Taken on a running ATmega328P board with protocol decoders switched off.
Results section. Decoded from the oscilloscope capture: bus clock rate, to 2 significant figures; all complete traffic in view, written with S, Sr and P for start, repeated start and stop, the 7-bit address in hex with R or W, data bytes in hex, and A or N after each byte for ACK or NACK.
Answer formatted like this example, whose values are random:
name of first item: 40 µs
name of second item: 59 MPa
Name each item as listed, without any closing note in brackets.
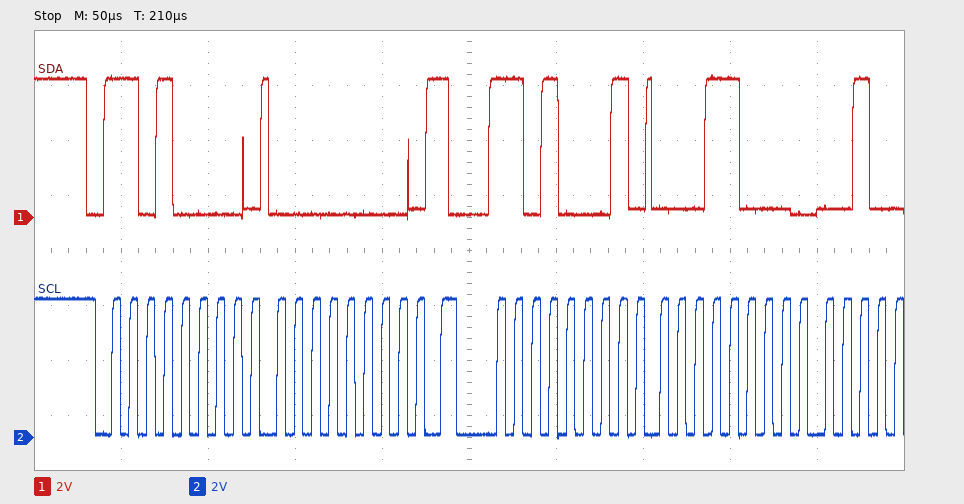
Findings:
bus clock rate, to 2 significant figures: 100 kHz
all complete traffic in view, written with S, Sr and P for start, repeated start and stop, the 7-bit address in hex with R or W, data bytes in hex, and A or N after each byte for ACK or NACK: S 68W A 00 A Sr 68R A 18 A
